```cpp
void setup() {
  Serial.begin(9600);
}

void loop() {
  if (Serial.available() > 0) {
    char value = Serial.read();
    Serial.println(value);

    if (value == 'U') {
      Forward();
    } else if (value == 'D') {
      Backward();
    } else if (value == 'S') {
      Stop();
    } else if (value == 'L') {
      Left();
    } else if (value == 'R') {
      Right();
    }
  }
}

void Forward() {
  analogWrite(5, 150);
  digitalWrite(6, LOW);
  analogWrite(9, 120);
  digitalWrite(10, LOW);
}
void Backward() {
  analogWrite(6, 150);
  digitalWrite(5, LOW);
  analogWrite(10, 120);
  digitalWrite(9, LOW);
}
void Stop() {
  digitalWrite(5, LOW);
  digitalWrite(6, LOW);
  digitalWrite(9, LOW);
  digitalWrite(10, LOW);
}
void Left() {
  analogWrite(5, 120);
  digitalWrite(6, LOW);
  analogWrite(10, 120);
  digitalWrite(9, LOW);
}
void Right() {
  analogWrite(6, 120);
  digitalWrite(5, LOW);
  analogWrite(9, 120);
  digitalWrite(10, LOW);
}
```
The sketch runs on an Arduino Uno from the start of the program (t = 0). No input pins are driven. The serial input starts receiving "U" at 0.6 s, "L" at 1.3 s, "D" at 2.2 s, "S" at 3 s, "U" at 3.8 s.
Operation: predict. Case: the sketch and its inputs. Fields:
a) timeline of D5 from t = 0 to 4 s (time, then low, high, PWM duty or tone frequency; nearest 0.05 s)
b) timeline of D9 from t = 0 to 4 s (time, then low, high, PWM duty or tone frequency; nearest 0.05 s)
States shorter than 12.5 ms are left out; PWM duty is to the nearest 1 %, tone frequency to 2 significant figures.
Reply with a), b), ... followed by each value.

a) 0.6 s PWM 59 %; 1.3 s PWM 47 %; 2.2 s low; 3.8 s PWM 59 %
b) 0.6 s PWM 47 %; 1.3 s low; 3.8 s PWM 47 %
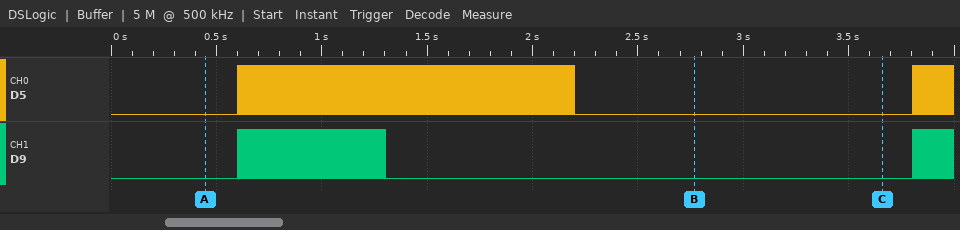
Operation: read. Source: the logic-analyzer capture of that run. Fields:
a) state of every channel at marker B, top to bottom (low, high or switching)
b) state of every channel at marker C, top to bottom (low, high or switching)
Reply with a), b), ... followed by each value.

a) D5 low, D9 low
b) D5 low, D9 low
